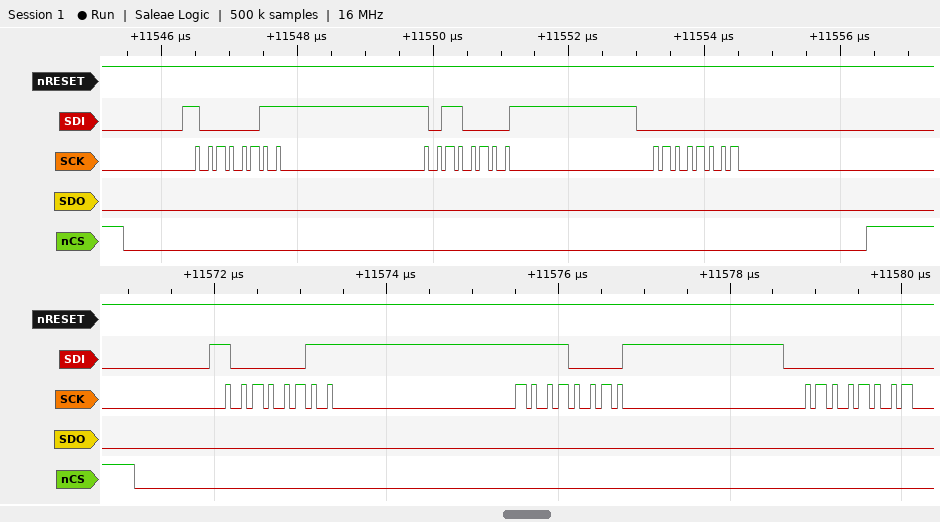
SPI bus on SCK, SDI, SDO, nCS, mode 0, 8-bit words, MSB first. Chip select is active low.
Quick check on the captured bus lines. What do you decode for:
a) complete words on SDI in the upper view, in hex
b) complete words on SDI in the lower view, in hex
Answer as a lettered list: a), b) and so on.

a) 83, B0, 00
b) 83, F0, 00
